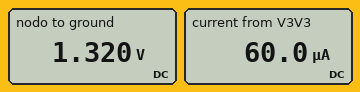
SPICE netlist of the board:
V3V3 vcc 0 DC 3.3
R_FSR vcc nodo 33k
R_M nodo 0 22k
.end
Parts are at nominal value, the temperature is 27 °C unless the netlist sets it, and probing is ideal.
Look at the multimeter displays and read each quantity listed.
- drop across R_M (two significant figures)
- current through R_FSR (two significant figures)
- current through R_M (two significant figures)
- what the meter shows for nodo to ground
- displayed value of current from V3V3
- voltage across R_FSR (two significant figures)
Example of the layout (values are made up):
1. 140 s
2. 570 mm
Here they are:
1. 1.3 V
2. 60 µA
3. 60 µA
4. 1.320 V
5. 60.0 µA
6. 2.0 V
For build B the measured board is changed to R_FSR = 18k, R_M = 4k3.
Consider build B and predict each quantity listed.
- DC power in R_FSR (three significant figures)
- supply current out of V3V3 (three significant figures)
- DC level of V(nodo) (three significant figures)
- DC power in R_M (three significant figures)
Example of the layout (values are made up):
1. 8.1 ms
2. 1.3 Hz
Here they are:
1. 394 µW
2. 148 µA
3. 636 mV
4. 94.2 µW
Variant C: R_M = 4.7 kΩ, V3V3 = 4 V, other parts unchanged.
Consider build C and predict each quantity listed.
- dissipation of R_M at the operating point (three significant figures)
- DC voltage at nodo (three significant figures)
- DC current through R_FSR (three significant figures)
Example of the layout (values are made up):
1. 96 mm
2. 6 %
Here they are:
1. 52.9 µW
2. 499 mV
3. 106 µA
